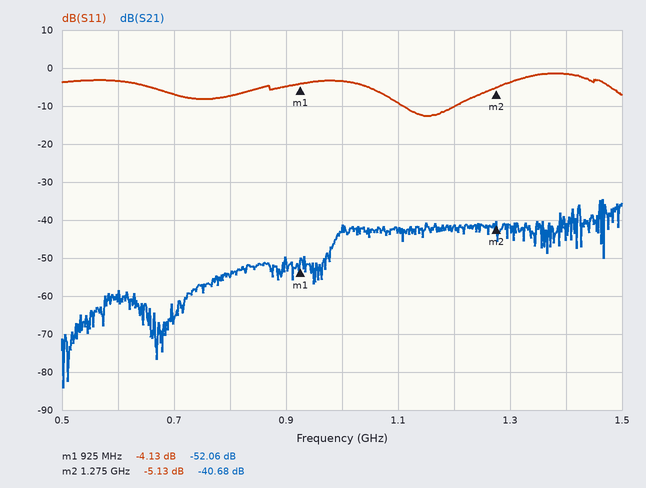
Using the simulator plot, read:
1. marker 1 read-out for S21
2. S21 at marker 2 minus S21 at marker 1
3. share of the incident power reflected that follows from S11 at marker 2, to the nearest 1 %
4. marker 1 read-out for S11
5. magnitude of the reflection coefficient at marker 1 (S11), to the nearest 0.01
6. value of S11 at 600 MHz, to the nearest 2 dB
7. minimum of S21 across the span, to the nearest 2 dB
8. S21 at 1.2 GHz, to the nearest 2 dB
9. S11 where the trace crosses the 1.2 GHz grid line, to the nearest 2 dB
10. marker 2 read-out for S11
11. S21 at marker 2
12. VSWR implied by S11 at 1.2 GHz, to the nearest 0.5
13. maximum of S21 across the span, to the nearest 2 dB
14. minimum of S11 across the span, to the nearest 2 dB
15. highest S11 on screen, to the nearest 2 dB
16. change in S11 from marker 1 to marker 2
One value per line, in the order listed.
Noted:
-52.06 dB
11.38 dB
31 %
-4.13 dB
0.62
-4 dB
-84 dB
-42 dB
-10 dB
-5.13 dB
-40.68 dB
2.0
-34 dB
-12 dB
-2 dB
-1.00 dB
